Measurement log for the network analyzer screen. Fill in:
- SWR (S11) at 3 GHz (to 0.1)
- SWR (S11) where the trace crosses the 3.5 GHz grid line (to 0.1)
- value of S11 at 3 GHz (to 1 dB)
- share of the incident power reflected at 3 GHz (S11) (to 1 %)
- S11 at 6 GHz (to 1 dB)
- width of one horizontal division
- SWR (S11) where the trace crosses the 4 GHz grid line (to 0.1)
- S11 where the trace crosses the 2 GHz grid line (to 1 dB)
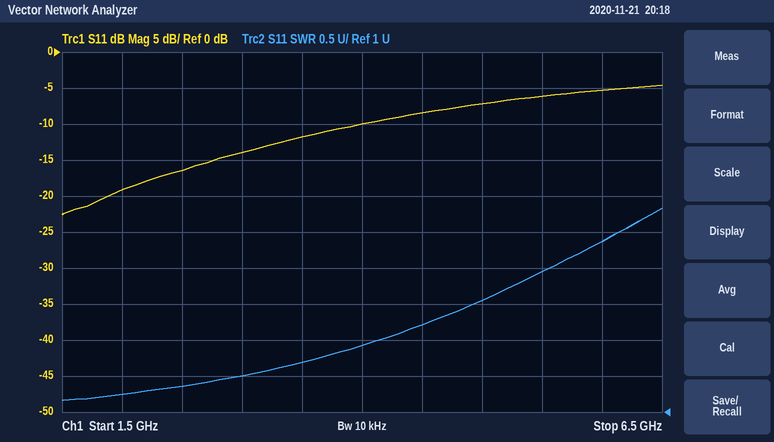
1.5
1.7
-14 dB
4 %
-5 dB
500 MHz
1.9
-19 dB
